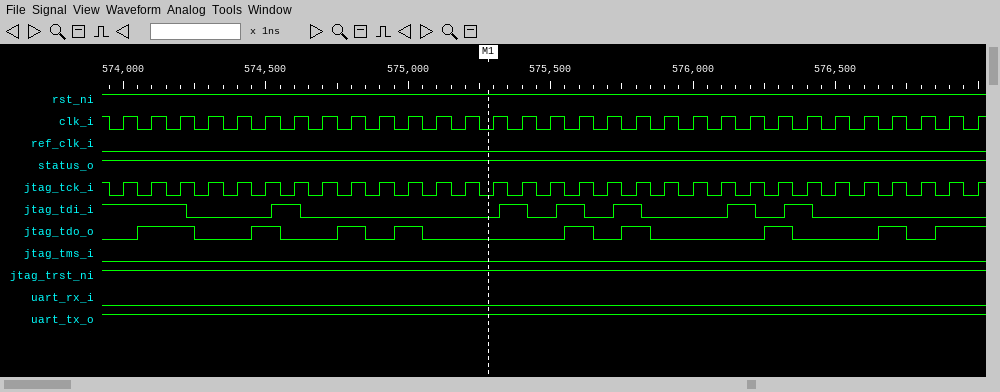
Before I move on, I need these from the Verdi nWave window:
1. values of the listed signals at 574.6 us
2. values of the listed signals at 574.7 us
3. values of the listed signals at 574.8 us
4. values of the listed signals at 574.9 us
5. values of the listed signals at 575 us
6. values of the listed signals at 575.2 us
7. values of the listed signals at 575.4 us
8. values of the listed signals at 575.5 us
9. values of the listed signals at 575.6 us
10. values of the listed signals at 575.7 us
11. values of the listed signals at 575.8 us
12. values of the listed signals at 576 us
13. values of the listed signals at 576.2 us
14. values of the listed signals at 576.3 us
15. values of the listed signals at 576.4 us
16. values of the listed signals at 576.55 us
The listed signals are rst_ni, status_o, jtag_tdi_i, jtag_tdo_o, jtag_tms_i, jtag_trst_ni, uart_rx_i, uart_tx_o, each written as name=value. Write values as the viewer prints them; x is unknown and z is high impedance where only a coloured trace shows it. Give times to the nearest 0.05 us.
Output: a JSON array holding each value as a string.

["rst_ni=1, status_o=1, jtag_tdi_i=1, jtag_tdo_o=0, jtag_tms_i=0, jtag_trst_ni=1, uart_rx_i=0, uart_tx_o=1", "rst_ni=1, status_o=1, jtag_tdi_i=0, jtag_tdo_o=0, jtag_tms_i=0, jtag_trst_ni=1, uart_rx_i=0, uart_tx_o=1", "rst_ni=1, status_o=1, jtag_tdi_i=0, jtag_tdo_o=1, jtag_tms_i=0, jtag_trst_ni=1, uart_rx_i=0, uart_tx_o=1", "rst_ni=1, status_o=1, jtag_tdi_i=0, jtag_tdo_o=0, jtag_tms_i=0, jtag_trst_ni=1, uart_rx_i=0, uart_tx_o=1", "rst_ni=1, status_o=1, jtag_tdi_i=0, jtag_tdo_o=1, jtag_tms_i=0, jtag_trst_ni=1, uart_rx_i=0, uart_tx_o=1", "rst_ni=1, status_o=1, jtag_tdi_i=0, jtag_tdo_o=0, jtag_tms_i=0, jtag_trst_ni=1, uart_rx_i=0, uart_tx_o=1", "rst_ni=1, status_o=1, jtag_tdi_i=1, jtag_tdo_o=0, jtag_tms_i=0, jtag_trst_ni=1, uart_rx_i=0, uart_tx_o=1", "rst_ni=1, status_o=1, jtag_tdi_i=0, jtag_tdo_o=0, jtag_tms_i=0, jtag_trst_ni=1, uart_rx_i=0, uart_tx_o=1", "rst_ni=1, status_o=1, jtag_tdi_i=1, jtag_tdo_o=1, jtag_tms_i=0, jtag_trst_ni=1, uart_rx_i=0, uart_tx_o=1", "rst_ni=1, status_o=1, jtag_tdi_i=0, jtag_tdo_o=0, jtag_tms_i=0, jtag_trst_ni=1, uart_rx_i=0, uart_tx_o=1", "rst_ni=1, status_o=1, jtag_tdi_i=1, jtag_tdo_o=1, jtag_tms_i=0, jtag_trst_ni=1, uart_rx_i=0, uart_tx_o=1", "rst_ni=1, status_o=1, jtag_tdi_i=0, jtag_tdo_o=0, jtag_tms_i=0, jtag_trst_ni=1, uart_rx_i=0, uart_tx_o=1", "rst_ni=1, status_o=1, jtag_tdi_i=1, jtag_tdo_o=0, jtag_tms_i=0, jtag_trst_ni=1, uart_rx_i=0, uart_tx_o=1", "rst_ni=1, status_o=1, jtag_tdi_i=0, jtag_tdo_o=1, jtag_tms_i=0, jtag_trst_ni=1, uart_rx_i=0, uart_tx_o=1", "rst_ni=1, status_o=1, jtag_tdi_i=1, jtag_tdo_o=0, jtag_tms_i=0, jtag_trst_ni=1, uart_rx_i=0, uart_tx_o=1", "rst_ni=1, status_o=1, jtag_tdi_i=0, jtag_tdo_o=0, jtag_tms_i=0, jtag_trst_ni=1, uart_rx_i=0, uart_tx_o=1"]
